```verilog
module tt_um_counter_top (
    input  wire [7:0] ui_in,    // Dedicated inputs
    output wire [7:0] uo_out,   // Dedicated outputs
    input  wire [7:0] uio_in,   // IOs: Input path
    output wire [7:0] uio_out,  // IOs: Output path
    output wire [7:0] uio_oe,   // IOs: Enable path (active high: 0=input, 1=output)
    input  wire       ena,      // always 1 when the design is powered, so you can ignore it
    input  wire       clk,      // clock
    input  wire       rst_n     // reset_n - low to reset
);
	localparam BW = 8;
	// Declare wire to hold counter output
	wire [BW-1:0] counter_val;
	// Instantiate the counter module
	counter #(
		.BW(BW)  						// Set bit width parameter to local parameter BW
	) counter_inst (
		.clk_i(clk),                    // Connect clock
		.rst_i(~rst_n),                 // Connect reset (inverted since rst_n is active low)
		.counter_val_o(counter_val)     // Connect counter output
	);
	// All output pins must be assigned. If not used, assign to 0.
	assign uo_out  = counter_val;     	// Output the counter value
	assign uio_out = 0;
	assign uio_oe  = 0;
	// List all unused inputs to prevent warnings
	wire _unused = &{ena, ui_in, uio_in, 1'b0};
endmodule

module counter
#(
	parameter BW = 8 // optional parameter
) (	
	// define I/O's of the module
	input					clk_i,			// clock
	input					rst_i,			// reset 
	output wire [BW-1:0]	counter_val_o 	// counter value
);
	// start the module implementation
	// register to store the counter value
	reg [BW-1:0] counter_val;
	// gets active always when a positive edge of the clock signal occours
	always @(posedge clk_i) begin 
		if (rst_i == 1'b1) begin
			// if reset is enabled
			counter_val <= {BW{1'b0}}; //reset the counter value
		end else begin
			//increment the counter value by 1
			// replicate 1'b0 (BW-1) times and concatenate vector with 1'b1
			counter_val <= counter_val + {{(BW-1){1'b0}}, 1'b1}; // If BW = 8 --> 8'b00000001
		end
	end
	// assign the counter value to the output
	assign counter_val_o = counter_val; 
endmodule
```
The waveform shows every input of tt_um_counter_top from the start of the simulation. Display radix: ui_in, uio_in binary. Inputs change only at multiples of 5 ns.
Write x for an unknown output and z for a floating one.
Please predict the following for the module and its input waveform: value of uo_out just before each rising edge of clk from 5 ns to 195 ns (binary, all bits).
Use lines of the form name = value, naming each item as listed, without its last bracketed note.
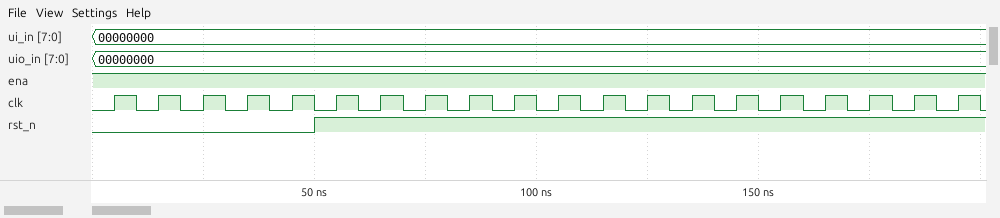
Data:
value of uo_out just before each rising edge of clk from 5 ns to 195 ns = x, 00000000, 00000000, 00000000, 00000000, 00000000, 00000001, 00000010, 00000011, 00000100, 00000101, 00000110, 00000111, 00001000, 00001001, 00001010, 00001011, 00001100, 00001101, 00001110
